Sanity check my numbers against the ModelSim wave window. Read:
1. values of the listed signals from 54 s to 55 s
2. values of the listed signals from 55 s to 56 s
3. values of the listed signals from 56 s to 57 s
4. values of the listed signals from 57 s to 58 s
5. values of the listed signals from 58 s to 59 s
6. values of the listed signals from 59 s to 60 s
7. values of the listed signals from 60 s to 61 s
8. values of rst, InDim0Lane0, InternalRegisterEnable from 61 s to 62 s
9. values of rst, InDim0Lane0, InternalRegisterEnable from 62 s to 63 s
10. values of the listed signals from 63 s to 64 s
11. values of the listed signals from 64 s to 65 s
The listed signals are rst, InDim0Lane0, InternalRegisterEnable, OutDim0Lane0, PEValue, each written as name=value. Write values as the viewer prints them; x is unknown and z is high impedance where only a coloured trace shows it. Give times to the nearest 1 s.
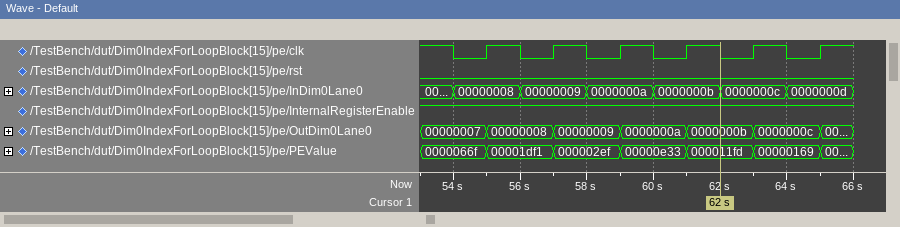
rst=0, InDim0Lane0=00000008, InternalRegisterEnable=1, OutDim0Lane0=00000007, PEValue=0000066f
rst=0, InDim0Lane0=00000008, InternalRegisterEnable=1, OutDim0Lane0=00000008, PEValue=00001df1
rst=0, InDim0Lane0=00000009, InternalRegisterEnable=1, OutDim0Lane0=00000008, PEValue=00001df1
rst=0, InDim0Lane0=00000009, InternalRegisterEnable=1, OutDim0Lane0=00000009, PEValue=000002ef
rst=0, InDim0Lane0=0000000a, InternalRegisterEnable=1, OutDim0Lane0=00000009, PEValue=000002ef
rst=0, InDim0Lane0=0000000a, InternalRegisterEnable=1, OutDim0Lane0=0000000a, PEValue=00000e33
rst=0, InDim0Lane0=0000000b, InternalRegisterEnable=1, OutDim0Lane0=0000000a, PEValue=00000e33
rst=0, InDim0Lane0=0000000b, InternalRegisterEnable=1
rst=0, InDim0Lane0=0000000c, InternalRegisterEnable=1
rst=0, InDim0Lane0=0000000c, InternalRegisterEnable=1, OutDim0Lane0=0000000c, PEValue=00000169
rst=0, InDim0Lane0=0000000d, InternalRegisterEnable=1, OutDim0Lane0=0000000c, PEValue=00000169
